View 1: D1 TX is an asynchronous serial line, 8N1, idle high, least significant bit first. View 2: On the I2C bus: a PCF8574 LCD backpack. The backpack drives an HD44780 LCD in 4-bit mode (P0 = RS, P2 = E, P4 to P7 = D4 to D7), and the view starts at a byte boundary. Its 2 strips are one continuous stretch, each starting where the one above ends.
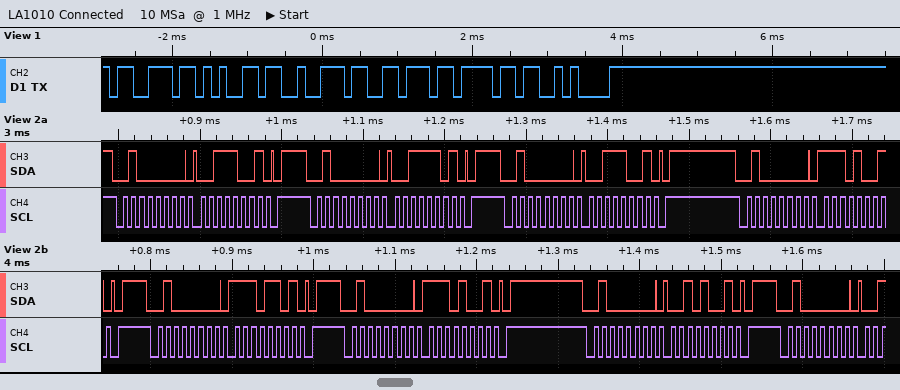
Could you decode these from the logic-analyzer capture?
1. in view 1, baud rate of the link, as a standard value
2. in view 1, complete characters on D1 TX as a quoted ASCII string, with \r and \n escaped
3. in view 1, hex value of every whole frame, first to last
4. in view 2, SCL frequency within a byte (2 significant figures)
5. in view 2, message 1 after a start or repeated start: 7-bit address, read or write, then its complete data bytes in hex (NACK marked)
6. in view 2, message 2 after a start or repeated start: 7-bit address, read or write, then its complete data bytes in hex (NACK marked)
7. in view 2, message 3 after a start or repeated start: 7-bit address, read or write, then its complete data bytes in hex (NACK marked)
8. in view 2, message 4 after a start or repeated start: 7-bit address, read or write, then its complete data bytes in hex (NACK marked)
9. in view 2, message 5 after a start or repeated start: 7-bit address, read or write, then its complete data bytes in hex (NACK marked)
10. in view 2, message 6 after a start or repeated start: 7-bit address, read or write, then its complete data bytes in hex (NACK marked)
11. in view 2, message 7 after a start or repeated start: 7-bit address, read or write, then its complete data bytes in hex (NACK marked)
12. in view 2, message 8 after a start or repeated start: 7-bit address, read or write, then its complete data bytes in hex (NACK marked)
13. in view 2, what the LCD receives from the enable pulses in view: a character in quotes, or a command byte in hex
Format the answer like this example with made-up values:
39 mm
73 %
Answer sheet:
9600 baud
"servo\n"
73 65 72 76 6F 0A
100 kHz
0x20 write: 39
0x20 write: 3D
0x20 write: 39
0x20 write: E9
0x20 write: ED
0x20 write: E9
0x20 write: 29
0x20 write
'>'
